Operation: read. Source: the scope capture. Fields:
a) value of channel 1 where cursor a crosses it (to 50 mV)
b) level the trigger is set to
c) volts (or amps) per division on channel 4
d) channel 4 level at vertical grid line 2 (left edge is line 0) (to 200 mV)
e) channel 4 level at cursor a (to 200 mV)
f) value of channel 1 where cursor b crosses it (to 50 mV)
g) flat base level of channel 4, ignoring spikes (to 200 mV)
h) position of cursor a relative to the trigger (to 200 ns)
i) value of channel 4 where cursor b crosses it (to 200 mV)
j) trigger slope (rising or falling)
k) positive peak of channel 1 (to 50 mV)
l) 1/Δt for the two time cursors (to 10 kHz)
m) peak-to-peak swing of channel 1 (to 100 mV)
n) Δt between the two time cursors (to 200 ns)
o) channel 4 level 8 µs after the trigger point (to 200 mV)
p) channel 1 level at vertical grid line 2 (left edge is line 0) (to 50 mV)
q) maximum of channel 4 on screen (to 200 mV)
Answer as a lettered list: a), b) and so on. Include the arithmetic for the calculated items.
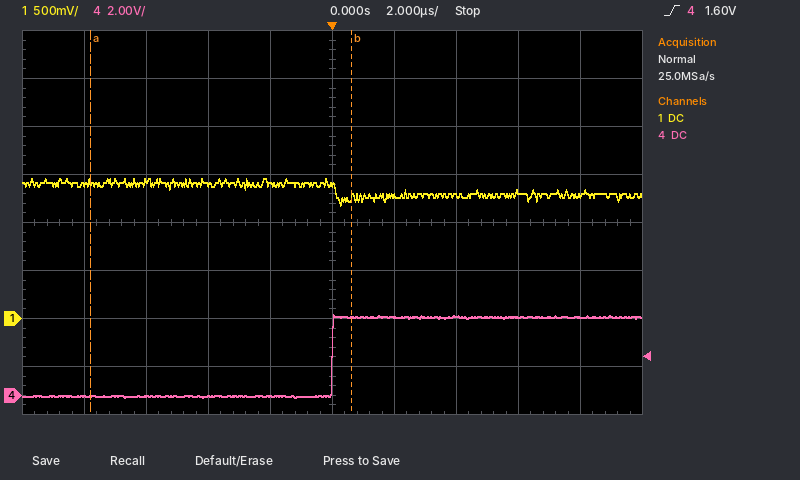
a) 1.40 V
b) 1.60 V
c) 2 V
d) 0.0 V
e) 0.0 V
f) 1.25 V
g) 0.0 V
h) -7.8 µs
i) 3.2 V
j) rising
k) 1.45 V
l) 1 / 8.4 µs ≈ 120 kHz
m) 300 mV
n) 8.4 µs
o) 3.2 V
p) 1.40 V
q) 3.4 V
